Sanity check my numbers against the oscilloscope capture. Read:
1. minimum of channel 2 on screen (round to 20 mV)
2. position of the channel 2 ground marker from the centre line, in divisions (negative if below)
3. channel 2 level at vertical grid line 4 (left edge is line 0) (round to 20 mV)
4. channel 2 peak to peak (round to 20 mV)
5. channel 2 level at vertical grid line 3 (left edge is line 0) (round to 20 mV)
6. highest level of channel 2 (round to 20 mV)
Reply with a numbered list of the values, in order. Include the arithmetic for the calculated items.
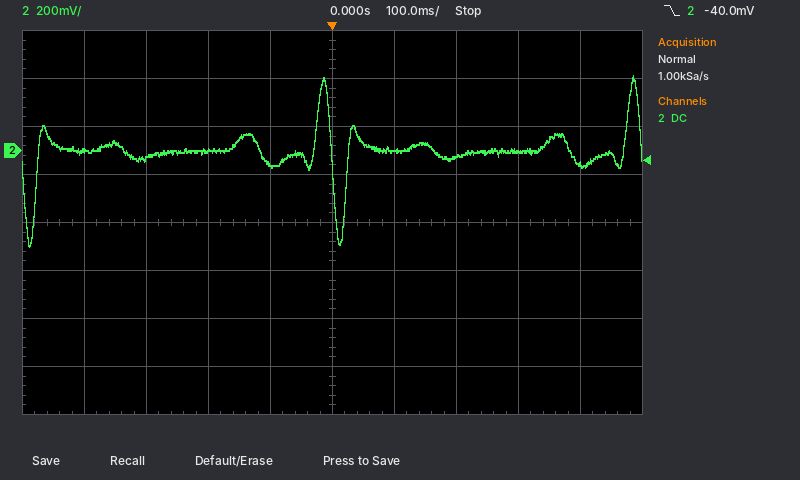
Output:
1. -400 mV
2. +1.5 div
3. -60 mV
4. 320 mV − (-400 mV) = 720 mV
5. 0 mV
6. 320 mV
